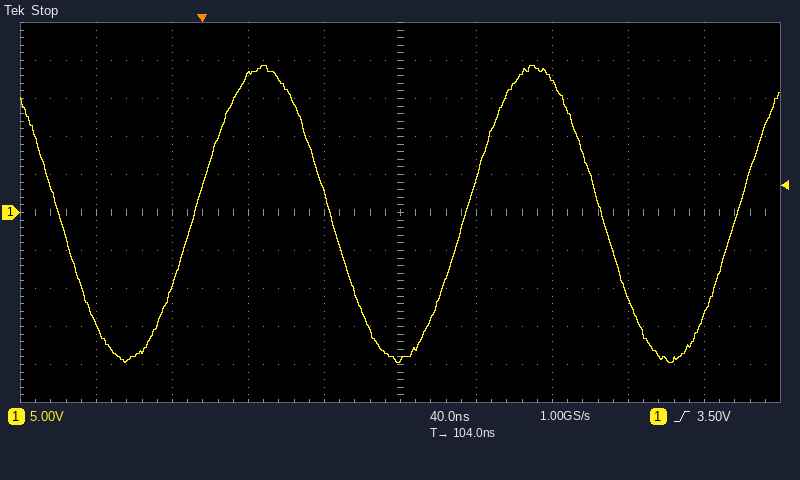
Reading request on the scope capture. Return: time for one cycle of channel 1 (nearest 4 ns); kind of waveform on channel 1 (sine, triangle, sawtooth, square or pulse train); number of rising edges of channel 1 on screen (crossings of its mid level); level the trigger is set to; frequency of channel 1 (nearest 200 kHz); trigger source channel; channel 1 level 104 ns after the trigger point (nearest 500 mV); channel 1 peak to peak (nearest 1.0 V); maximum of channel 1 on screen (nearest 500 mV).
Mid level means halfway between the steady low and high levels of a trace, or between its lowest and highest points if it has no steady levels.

144 ns
sine
3
3.50 V
7.0 MHz
channel 1
-19.5 V
39.0 V
19.5 V
